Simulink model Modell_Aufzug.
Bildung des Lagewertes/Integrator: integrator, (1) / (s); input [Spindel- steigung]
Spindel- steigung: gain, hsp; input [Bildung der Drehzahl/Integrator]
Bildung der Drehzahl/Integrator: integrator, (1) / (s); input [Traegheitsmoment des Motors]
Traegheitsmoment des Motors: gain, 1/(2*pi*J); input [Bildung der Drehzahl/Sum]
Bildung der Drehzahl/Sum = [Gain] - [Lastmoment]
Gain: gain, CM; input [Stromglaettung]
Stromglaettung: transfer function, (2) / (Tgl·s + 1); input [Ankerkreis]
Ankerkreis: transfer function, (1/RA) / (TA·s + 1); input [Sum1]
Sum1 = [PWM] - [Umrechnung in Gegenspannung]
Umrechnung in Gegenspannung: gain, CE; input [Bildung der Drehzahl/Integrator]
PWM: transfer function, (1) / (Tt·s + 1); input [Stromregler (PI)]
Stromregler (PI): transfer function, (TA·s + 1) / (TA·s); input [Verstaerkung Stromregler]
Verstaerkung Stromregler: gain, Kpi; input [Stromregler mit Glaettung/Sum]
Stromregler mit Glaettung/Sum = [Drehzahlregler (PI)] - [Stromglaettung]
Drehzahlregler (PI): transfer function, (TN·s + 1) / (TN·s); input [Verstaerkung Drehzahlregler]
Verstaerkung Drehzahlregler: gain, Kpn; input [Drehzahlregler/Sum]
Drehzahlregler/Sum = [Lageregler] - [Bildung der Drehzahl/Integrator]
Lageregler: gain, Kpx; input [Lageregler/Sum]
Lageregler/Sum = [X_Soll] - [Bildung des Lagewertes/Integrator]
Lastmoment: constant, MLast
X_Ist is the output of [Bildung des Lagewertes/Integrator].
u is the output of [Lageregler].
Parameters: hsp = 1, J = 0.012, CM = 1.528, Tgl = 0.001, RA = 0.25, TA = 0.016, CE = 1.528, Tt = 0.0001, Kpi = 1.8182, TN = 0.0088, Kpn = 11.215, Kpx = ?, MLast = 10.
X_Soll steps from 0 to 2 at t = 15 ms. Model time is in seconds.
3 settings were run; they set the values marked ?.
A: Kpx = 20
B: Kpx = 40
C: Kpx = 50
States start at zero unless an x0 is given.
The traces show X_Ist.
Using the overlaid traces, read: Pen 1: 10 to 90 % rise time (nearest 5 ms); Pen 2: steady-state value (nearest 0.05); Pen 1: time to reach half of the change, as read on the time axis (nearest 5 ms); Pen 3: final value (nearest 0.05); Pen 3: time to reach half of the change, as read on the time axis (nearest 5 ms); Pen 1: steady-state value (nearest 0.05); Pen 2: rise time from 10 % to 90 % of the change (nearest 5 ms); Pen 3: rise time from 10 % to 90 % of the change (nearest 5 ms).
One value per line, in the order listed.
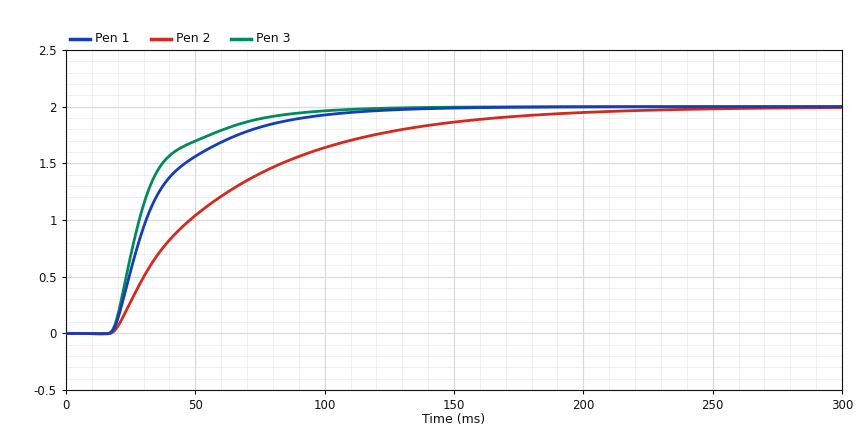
50 ms
2.00
30 ms
2.00
30 ms
2.00
105 ms
40 ms
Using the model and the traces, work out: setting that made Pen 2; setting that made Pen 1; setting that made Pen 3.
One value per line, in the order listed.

A
B
C
